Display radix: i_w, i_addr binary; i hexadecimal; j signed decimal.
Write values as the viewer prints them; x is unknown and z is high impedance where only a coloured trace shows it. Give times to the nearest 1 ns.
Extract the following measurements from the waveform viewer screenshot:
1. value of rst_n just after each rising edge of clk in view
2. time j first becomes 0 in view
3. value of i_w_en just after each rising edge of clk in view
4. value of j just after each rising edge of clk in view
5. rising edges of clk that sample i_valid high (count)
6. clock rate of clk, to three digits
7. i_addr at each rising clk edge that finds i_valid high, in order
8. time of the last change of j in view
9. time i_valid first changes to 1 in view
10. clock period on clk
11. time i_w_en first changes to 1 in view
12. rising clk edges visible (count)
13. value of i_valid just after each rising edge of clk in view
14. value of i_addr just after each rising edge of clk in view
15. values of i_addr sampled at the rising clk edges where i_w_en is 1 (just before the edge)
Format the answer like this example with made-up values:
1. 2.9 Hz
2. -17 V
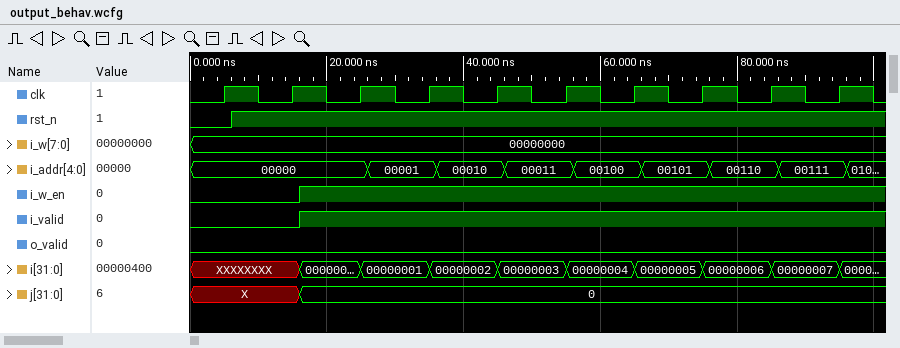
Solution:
1. 0 1 1 1 1 1 1 1 1 1
2. 16 ns
3. 0 0 1 1 1 1 1 1 1 1
4. X, X, 0, 0, 0, 0, 0, 0, 0, 0
5. 8
6. 100 MHz
7. 00000, 00001, 00010, 00011, 00100, 00101, 00110, 00111
8. 16 ns
9. 16 ns
10. 10 ns
11. 16 ns
12. 10
13. 0 0 1 1 1 1 1 1 1 1
14. 00000, 00000, 00000, 00001, 00010, 00011, 00100, 00101, 00110, 00111
15. 00000, 00001, 00010, 00011, 00100, 00101, 00110, 00111
